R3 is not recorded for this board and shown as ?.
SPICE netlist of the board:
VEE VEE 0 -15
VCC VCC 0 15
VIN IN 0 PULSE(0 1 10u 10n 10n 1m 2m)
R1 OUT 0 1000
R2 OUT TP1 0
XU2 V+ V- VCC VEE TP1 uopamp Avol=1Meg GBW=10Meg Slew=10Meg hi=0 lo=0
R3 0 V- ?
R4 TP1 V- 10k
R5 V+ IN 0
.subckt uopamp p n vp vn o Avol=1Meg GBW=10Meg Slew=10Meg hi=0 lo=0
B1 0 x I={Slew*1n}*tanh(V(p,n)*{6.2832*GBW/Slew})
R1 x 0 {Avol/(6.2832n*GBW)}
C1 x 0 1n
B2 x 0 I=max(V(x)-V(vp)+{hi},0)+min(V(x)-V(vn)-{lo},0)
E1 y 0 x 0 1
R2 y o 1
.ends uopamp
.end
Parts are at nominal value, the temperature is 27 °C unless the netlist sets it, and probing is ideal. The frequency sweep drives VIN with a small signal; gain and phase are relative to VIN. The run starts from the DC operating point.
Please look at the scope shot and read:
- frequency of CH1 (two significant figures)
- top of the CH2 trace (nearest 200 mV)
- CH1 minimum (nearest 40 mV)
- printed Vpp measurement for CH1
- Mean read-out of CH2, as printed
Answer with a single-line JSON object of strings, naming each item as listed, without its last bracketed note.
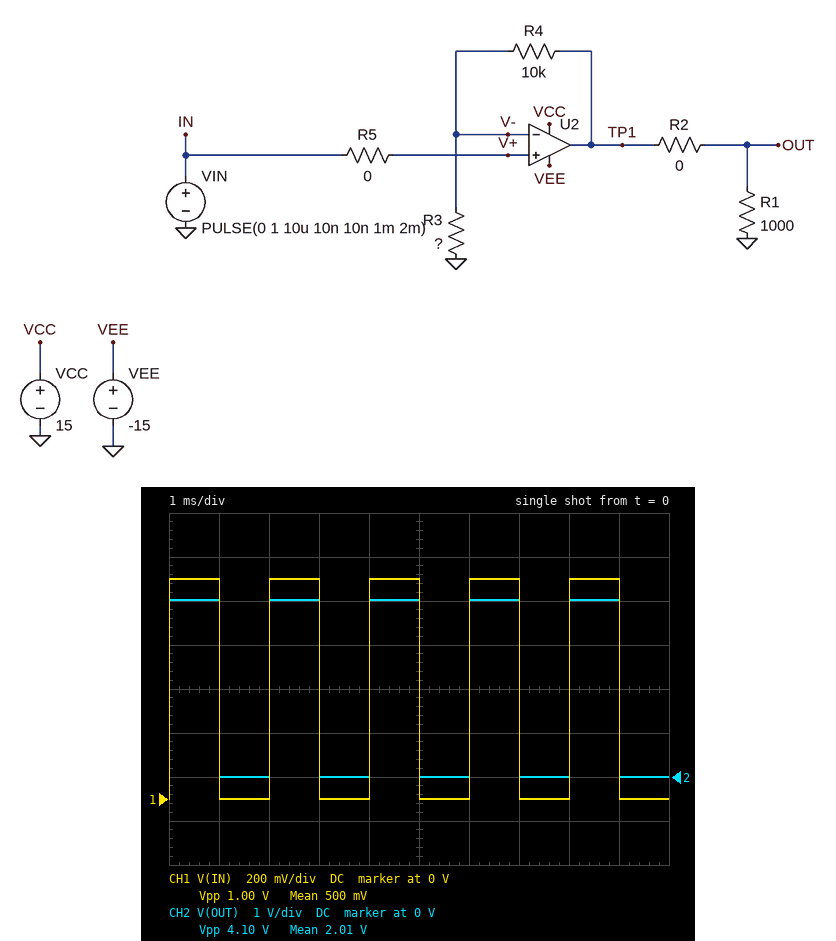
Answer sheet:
{"frequency of CH1": "500 Hz", "top of the CH2 trace": "4.0 V", "CH1 minimum": "0 V", "printed Vpp measurement for CH1": "1.00 V", "Mean read-out of CH2, as printed": "2.01 V"}
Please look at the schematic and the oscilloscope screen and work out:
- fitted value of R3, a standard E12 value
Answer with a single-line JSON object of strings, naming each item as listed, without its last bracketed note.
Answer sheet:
{"fitted value of R3, a standard E12 value": "3.3 kΩ"}
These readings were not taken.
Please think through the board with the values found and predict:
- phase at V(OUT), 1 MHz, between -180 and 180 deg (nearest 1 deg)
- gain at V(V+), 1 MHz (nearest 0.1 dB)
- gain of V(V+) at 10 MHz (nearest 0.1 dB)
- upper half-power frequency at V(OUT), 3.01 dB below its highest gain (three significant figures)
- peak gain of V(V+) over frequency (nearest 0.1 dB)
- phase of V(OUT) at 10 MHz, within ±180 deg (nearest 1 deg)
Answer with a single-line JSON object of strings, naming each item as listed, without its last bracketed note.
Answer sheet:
{"phase at V(OUT), 1 MHz, between -180 and 180 deg": "-22 deg", "gain at V(V+), 1 MHz": "0 dB", "gain of V(V+) at 10 MHz": "0 dB", "upper half-power frequency at V(OUT), 3.01 dB below its highest gain": "2.48 MHz", "peak gain of V(V+) over frequency": "0 dB", "phase of V(OUT) at 10 MHz, within ±180 deg": "-76 deg"}
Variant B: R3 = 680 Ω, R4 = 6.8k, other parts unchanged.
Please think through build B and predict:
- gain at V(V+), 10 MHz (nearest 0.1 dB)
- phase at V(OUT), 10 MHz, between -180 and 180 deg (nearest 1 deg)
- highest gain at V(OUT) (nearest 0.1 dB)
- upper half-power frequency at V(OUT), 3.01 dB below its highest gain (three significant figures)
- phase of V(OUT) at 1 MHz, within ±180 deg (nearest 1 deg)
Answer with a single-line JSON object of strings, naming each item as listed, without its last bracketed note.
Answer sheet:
{"gain at V(V+), 10 MHz": "0 dB", "phase at V(OUT), 10 MHz, between -180 and 180 deg": "-85 deg", "highest gain at V(OUT)": "20.8 dB", "upper half-power frequency at V(OUT), 3.01 dB below its highest gain": "908 kHz", "phase of V(OUT) at 1 MHz, within ±180 deg": "-48 deg"}
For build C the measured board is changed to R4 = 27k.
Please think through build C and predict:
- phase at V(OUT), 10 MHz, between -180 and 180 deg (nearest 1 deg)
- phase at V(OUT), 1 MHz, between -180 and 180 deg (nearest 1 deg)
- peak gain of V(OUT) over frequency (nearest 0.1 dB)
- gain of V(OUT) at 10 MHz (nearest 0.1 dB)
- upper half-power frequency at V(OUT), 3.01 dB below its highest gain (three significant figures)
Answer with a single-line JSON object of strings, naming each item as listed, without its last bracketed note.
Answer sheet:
{"phase at V(OUT), 10 MHz, between -180 and 180 deg": "-84 deg", "phase at V(OUT), 1 MHz, between -180 and 180 deg": "-43 deg", "peak gain of V(OUT) over frequency": "19.3 dB", "gain of V(OUT) at 10 MHz": "-0.1 dB", "upper half-power frequency at V(OUT), 3.01 dB below its highest gain": "1.09 MHz"}
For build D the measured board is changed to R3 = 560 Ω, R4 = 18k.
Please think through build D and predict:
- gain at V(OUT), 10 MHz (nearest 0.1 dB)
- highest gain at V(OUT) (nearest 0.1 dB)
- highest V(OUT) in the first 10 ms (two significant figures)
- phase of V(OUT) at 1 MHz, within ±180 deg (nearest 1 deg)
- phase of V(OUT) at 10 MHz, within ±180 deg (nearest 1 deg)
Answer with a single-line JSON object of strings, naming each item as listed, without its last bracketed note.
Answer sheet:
{"gain at V(OUT), 10 MHz": "0 dB", "highest gain at V(OUT)": "30.4 dB", "highest V(OUT) in the first 10 ms": "15 V", "phase of V(OUT) at 1 MHz, within ±180 deg": "-73 deg", "phase of V(OUT) at 10 MHz, within ±180 deg": "-88 deg"}
